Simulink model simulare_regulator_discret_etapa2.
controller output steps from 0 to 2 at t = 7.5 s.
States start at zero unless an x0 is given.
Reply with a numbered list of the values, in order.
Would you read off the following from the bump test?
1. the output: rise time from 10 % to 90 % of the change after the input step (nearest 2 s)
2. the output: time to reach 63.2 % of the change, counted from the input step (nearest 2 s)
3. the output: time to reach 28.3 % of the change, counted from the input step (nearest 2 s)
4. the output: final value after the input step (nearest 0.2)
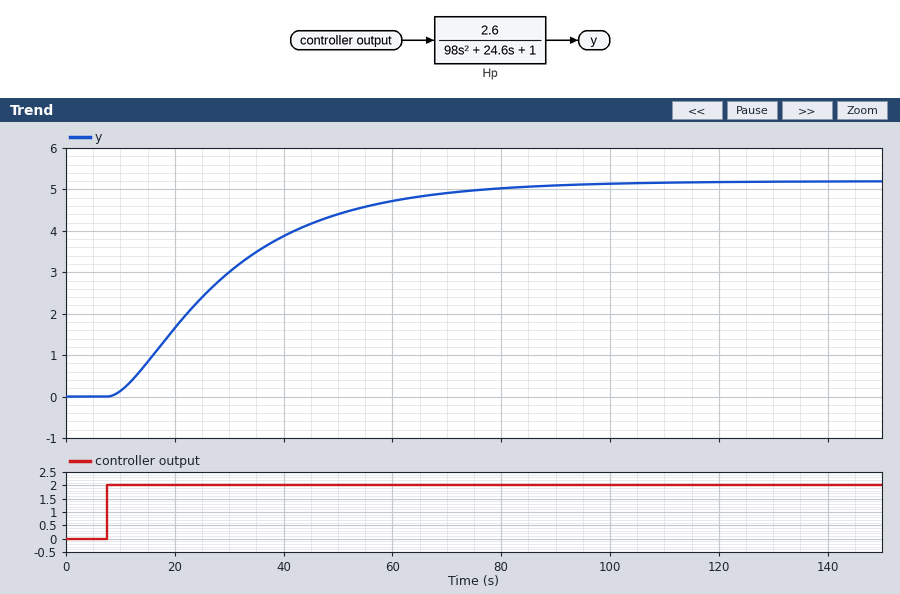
1. 46 s
2. 26 s
3. 12 s
4. 5.2
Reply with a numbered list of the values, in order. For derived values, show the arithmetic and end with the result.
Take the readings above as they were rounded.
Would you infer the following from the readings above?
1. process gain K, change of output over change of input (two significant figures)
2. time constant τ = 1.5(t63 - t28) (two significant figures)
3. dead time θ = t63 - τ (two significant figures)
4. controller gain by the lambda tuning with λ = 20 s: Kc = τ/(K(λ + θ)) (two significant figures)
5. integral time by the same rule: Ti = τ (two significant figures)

1. (5.2 - 0) / 2 = 2.6
2. 1.5 × (26 - 12) = 21 s
3. 26 - 21 = 5.0 s
4. 21 / (2.6 × (20 + 5)) = 0.32
5. 21 s
